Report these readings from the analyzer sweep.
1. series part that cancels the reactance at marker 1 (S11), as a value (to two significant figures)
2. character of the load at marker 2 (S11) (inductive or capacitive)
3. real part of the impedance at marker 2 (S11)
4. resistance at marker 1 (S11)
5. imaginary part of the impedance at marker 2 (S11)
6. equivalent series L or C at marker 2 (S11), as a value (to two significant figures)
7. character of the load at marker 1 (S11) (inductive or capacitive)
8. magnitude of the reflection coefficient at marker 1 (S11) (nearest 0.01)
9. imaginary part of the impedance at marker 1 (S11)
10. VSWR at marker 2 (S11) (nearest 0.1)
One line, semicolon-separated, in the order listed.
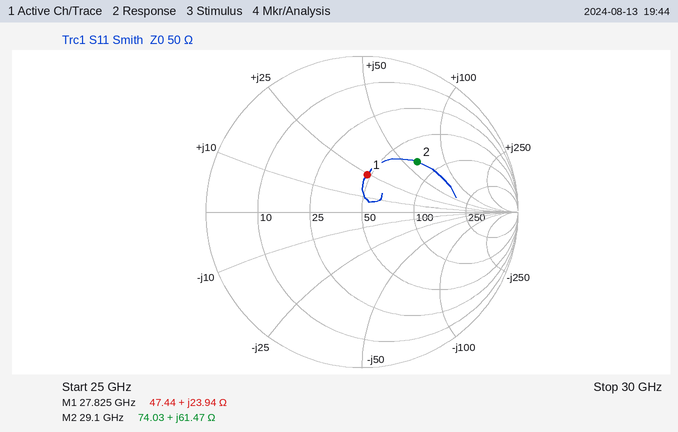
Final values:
240 fF; inductive; 74.03 Ω; 47.44 Ω; +61.47 Ω; 340 pH; inductive; 0.24; +23.94 Ω; 2.8
